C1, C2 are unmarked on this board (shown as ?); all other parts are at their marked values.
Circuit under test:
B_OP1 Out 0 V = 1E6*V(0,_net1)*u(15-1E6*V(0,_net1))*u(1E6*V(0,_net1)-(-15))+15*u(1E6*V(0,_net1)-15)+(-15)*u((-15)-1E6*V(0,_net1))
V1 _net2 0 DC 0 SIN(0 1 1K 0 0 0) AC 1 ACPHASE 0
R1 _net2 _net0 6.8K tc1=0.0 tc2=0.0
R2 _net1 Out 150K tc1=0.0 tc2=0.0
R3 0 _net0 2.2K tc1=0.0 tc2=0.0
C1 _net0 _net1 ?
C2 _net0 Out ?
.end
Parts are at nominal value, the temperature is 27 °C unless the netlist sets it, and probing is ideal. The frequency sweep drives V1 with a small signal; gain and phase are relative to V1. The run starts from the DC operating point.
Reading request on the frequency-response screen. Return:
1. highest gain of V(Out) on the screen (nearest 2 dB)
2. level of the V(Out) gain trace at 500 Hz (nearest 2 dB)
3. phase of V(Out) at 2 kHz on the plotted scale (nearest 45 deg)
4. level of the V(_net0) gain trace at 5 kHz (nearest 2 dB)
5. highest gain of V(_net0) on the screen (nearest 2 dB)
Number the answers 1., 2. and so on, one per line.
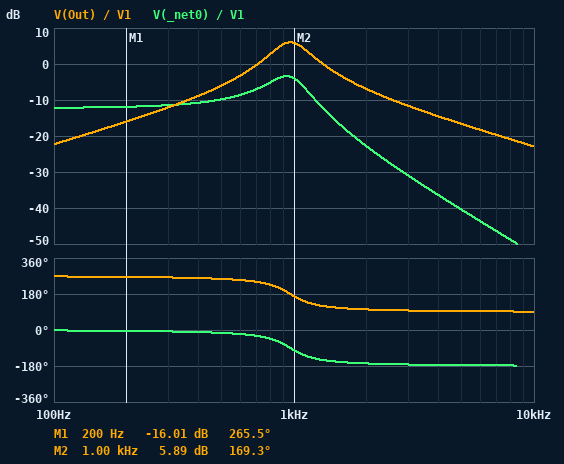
1. 6 dB
2. -6 dB
3. 90 deg
4. -40 dB
5. -4 dB
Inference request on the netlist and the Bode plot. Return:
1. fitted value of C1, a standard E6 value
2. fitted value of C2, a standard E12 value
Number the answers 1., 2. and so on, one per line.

1. 3.3 nF
2. 33 nF
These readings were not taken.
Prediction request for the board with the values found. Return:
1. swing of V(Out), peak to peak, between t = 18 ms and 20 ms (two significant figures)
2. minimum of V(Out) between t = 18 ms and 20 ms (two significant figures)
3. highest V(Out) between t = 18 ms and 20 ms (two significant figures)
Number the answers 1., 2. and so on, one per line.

1. 3.9 V
2. -2.0 V
3. 2.0 V
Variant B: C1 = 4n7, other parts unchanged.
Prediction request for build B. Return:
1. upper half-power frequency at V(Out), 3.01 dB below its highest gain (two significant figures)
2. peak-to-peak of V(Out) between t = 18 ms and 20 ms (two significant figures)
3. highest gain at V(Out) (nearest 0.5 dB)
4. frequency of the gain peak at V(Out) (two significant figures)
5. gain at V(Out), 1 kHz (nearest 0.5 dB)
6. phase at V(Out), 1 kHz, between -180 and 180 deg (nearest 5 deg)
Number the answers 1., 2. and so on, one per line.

1. 950 Hz
2. 3.3 V
3. 9.0 dB
4. 810 Hz
5. 4.5 dB
6. 125 deg
